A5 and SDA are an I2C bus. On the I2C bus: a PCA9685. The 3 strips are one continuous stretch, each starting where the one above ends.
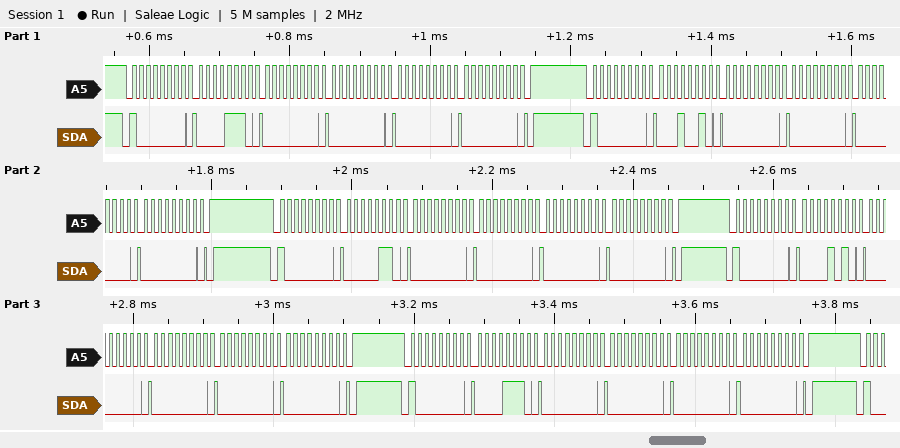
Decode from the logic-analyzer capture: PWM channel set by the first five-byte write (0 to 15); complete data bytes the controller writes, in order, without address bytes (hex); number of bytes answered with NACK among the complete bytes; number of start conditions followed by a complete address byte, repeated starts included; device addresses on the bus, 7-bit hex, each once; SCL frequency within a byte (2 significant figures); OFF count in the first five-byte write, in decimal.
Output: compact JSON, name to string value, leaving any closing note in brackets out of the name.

{"PWM channel set by the first five-byte write": "2", "complete data bytes the controller writes, in order, without address bytes": "0E 00 00 00 00 12 00 00 00 00 06 00 00 00 00 0A 00 00 00 00 0E 00 00 00 00", "number of bytes answered with NACK among the complete bytes": "0", "number of start conditions followed by a complete address byte, repeated starts included": "5", "device addresses on the bus, 7-bit hex, each once": "0x40", "SCL frequency within a byte": "100 kHz", "OFF count in the first five-byte write, in decimal": "0"}
